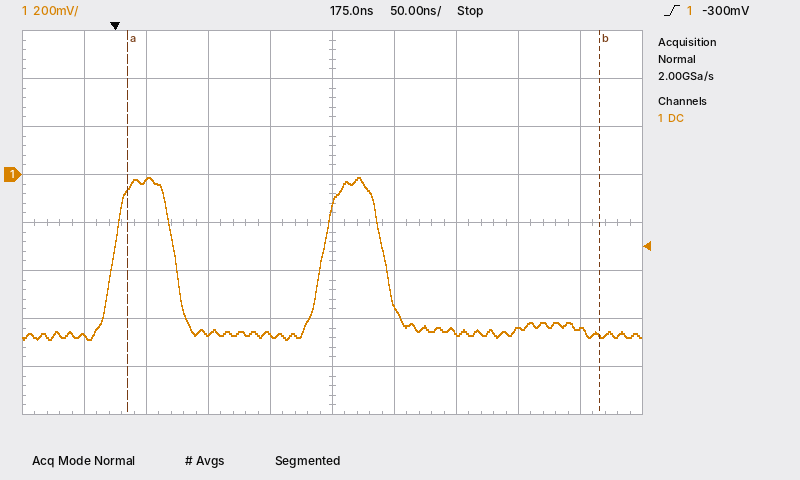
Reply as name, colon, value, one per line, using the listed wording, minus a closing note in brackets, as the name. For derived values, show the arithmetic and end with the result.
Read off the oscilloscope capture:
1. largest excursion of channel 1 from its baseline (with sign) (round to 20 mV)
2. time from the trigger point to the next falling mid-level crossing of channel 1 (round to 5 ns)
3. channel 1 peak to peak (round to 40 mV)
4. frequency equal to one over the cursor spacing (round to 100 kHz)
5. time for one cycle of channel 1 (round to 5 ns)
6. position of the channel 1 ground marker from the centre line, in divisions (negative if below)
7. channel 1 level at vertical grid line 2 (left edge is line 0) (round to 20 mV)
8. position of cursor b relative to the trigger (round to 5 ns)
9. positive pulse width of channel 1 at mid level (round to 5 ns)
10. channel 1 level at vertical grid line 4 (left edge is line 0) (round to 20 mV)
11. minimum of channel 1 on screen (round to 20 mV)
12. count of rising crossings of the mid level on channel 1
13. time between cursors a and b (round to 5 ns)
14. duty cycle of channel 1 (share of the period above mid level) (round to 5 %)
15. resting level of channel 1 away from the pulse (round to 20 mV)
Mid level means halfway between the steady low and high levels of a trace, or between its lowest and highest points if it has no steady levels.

largest excursion of channel 1 from its baseline (with sign): +640 mV
time from the trigger point to the next falling mid-level crossing of channel 1: 50 ns
channel 1 peak to peak: 680 mV
frequency equal to one over the cursor spacing: 1 / 380 ns ≈ 2.6 MHz
time for one cycle of channel 1: 170 ns
position of the channel 1 ground marker from the centre line, in divisions: +1.0 div
channel 1 level at vertical grid line 2 (left edge is line 0): -20 mV
position of cursor b relative to the trigger: +390 ns
positive pulse width of channel 1 at mid level: 50 ns
channel 1 level at vertical grid line 4 (left edge is line 0): -660 mV
minimum of channel 1 on screen: -680 mV
count of rising crossings of the mid level on channel 1: 2
time between cursors a and b: 380 ns
duty cycle of channel 1 (share of the period above mid level): 50 ns / 170 ns ≈ 29.4 %, so 30 % to the nearest 5 %
resting level of channel 1 away from the pulse: -660 mV
